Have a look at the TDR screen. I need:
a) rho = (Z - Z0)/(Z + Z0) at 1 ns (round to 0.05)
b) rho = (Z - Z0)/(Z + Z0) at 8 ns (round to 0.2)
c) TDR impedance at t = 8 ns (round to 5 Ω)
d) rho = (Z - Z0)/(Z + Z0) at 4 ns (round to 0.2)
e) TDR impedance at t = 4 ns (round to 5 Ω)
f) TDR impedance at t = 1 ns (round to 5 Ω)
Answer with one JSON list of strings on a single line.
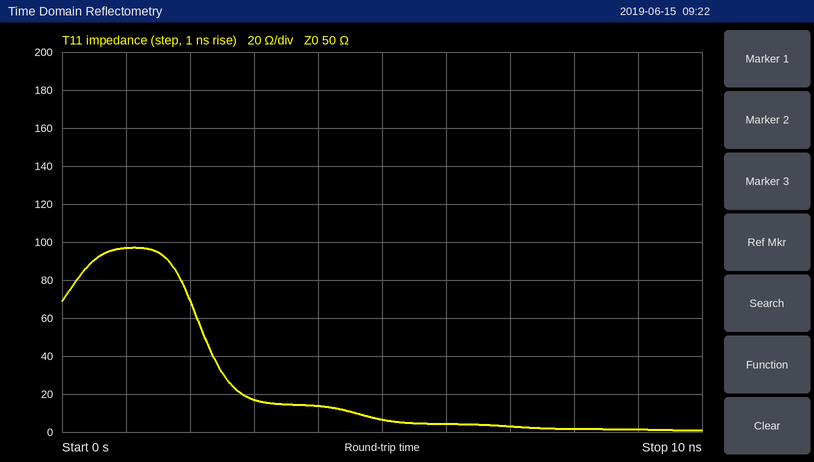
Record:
["+0.30", "-1.0", "0 Ω", "-0.6", "15 Ω", "95 Ω"]
